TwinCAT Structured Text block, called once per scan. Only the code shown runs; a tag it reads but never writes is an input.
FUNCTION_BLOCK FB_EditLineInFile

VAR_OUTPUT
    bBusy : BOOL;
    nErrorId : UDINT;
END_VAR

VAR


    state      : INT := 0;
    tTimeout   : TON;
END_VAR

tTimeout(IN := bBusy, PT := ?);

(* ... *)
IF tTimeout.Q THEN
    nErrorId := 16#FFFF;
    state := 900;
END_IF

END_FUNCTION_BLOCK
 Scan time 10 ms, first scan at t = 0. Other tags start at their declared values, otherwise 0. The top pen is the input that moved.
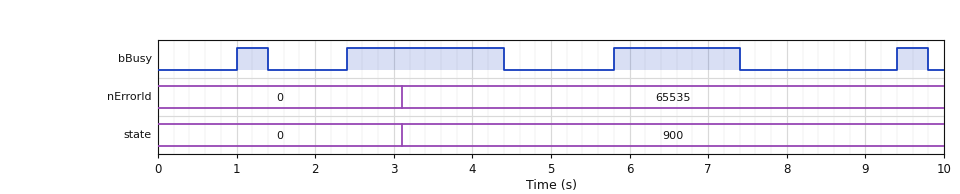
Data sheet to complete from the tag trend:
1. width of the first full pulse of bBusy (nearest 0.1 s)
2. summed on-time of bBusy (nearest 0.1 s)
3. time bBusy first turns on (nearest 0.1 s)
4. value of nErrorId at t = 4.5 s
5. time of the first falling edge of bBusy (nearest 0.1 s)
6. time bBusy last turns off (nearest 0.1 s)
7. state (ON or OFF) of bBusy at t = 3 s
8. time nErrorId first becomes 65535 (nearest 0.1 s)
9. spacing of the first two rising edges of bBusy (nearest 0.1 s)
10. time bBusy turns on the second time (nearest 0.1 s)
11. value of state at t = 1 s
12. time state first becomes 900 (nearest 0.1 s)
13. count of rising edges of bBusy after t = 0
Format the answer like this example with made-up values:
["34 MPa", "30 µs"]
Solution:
["0.4 s", "4.4 s", "1.0 s", "65535", "1.4 s", "9.8 s", "ON", "3.1 s", "1.4 s", "2.4 s", "0", "3.1 s", "4"]
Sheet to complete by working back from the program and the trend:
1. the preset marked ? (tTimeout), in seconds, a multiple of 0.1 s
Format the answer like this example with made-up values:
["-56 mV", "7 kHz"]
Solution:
["0.7 s"]
